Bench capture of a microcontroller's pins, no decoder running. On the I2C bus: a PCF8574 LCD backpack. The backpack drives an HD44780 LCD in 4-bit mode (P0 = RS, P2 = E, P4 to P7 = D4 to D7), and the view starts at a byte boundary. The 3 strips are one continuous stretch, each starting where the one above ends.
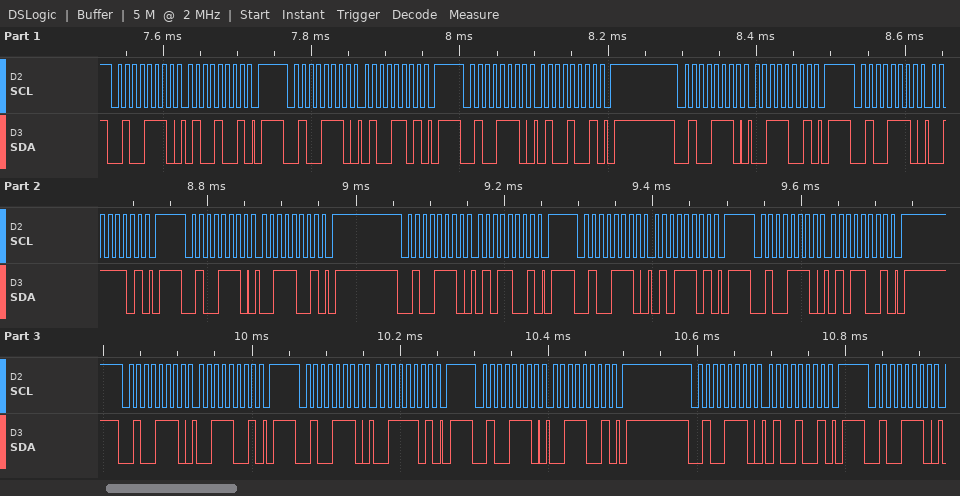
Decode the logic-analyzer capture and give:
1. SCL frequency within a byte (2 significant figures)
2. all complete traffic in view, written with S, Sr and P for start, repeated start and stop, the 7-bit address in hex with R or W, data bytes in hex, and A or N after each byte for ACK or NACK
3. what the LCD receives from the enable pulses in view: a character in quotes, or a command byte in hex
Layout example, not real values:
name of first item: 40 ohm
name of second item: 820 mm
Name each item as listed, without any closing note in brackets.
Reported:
SCL frequency within a byte: 100 kHz
all complete traffic in view, written with S, Sr and P for start, repeated start and stop, the 7-bit address in hex with R or W, data bytes in hex, and A or N after each byte for ACK or NACK: S 27W A 49 A P S 27W A 4D A P S 27W A 49 A P S 27W A 39 A P S 27W A 3D A P S 27W A 39 A P S 27W A 59 A P S 27W A 5D A P S 27W A 59 A P S 27W A 39 A P S 27W A 3D A P S 27W A 39 A P S 27W A 49 A P S 27W A
what the LCD receives from the enable pulses in view: a character in quotes, or a command byte in hex: 'C' 'S'
